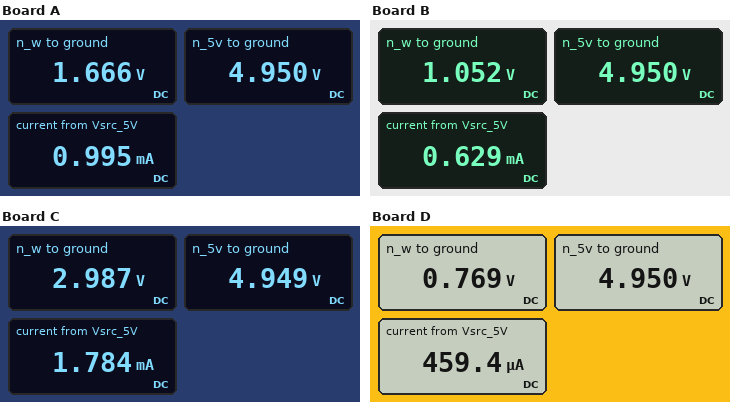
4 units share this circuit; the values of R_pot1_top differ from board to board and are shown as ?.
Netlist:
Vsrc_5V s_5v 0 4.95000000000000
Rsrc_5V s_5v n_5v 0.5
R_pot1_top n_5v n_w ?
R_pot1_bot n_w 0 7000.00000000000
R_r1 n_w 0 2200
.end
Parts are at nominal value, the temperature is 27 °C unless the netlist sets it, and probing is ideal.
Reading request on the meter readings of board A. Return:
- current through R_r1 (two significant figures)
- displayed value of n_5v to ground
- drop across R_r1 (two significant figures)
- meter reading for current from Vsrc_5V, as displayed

760 µA
4.950 V
1.7 V
0.995 mA
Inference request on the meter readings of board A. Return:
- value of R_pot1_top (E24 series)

3.3 kΩ
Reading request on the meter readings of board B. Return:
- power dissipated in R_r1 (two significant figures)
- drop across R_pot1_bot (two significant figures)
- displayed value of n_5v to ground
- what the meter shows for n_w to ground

500 µW
1.1 V
4.950 V
1.052 V
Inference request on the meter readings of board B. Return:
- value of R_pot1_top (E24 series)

6.2 kΩ
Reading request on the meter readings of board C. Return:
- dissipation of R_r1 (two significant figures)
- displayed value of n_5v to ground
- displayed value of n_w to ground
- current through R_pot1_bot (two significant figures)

4.1 mW
4.949 V
2.987 V
430 µA
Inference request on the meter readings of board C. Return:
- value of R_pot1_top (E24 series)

1.1 kΩ
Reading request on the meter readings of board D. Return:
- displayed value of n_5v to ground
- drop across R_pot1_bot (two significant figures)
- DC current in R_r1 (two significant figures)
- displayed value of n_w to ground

4.950 V
770 mV
350 µA
0.769 V
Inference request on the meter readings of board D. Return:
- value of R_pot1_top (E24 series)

9.1 kΩ
